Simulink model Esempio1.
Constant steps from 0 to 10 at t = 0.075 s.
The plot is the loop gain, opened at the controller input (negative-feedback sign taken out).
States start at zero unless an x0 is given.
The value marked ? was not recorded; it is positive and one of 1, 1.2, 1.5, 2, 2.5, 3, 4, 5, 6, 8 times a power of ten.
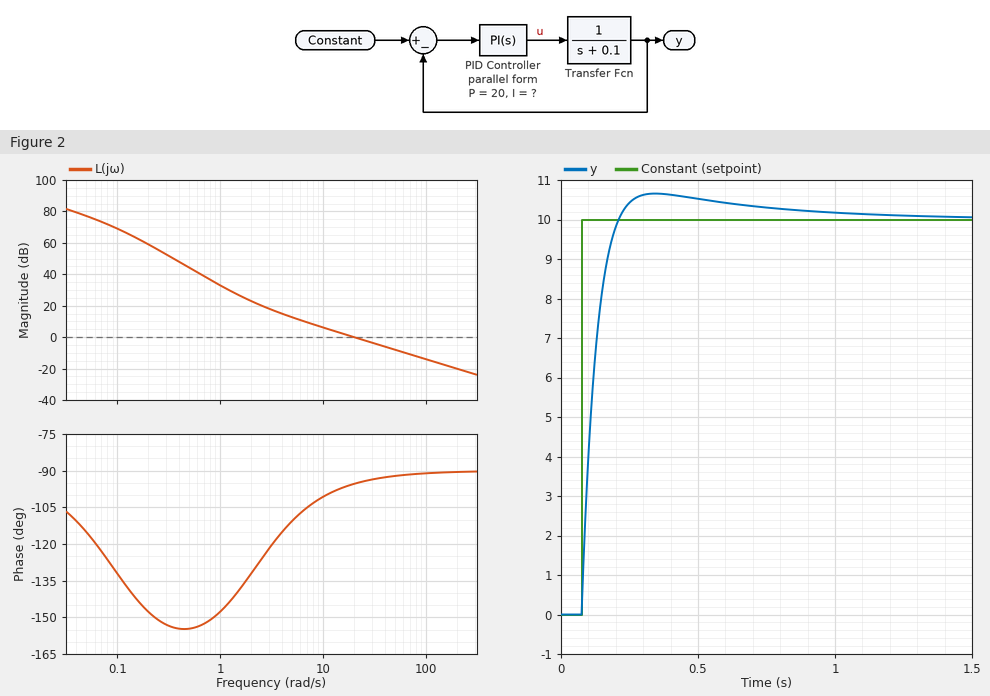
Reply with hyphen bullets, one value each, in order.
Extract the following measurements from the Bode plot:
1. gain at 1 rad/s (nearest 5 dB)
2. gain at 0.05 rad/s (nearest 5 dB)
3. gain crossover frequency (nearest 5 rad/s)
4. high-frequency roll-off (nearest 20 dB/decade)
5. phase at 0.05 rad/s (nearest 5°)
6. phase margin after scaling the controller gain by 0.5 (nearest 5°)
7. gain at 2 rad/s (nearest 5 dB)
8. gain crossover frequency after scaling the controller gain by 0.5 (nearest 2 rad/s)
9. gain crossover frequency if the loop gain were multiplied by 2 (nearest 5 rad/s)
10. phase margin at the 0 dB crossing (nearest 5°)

- 35 dB
- 75 dB
- 20 rad/s
- -20 dB/decade
- -115°
- 80°
- 25 dB
- 10 rad/s
- 40 rad/s
- 85°
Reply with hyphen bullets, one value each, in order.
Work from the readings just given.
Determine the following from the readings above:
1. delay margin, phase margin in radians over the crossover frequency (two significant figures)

- 0.074 s
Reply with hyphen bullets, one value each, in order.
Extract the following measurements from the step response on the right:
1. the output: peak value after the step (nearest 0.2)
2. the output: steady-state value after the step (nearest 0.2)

- 10.6
- 10.0
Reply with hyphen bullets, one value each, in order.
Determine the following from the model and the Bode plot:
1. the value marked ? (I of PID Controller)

- 40
